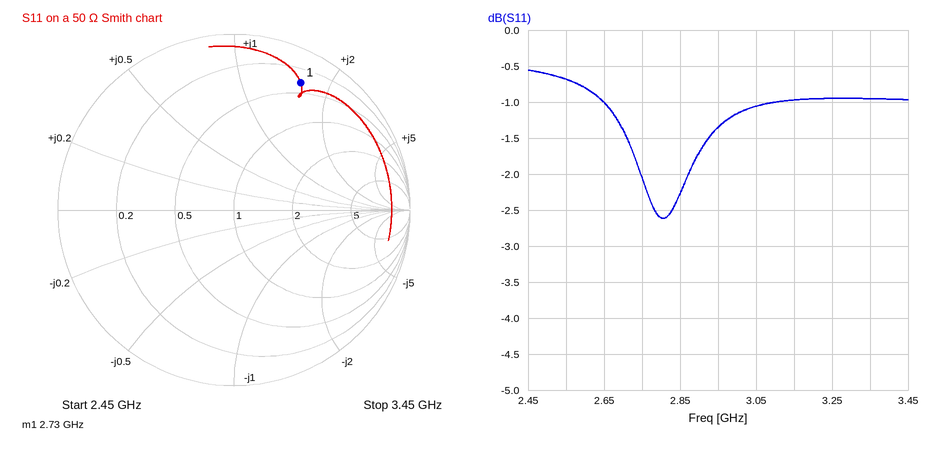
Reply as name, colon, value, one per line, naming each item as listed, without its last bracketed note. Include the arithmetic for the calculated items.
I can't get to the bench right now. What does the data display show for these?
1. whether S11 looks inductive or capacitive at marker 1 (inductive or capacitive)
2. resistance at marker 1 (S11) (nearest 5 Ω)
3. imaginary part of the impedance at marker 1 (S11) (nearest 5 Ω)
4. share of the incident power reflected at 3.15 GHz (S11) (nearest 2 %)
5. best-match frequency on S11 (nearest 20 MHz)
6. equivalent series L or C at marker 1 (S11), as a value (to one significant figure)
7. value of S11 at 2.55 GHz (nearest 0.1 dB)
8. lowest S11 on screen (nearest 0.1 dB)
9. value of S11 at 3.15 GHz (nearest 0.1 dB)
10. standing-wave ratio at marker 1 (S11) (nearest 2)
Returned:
whether S11 looks inductive or capacitive at marker 1: inductive
resistance at marker 1 (S11): 20 Ω
imaginary part of the impedance at marker 1 (S11): +80 Ω
share of the incident power reflected at 3.15 GHz (S11): 10^(-1/10) ≈ 79.4 %, so 80 % to the nearest 2 %
best-match frequency on S11: 2.80 GHz
equivalent series L or C at marker 1 (S11), as a value: L = 80 Ω/(2π × 2.73 GHz) ≈ 5 nH
value of S11 at 2.55 GHz: -0.7 dB
lowest S11 on screen: -2.6 dB
value of S11 at 3.15 GHz: -1.0 dB
standing-wave ratio at marker 1 (S11): 10
